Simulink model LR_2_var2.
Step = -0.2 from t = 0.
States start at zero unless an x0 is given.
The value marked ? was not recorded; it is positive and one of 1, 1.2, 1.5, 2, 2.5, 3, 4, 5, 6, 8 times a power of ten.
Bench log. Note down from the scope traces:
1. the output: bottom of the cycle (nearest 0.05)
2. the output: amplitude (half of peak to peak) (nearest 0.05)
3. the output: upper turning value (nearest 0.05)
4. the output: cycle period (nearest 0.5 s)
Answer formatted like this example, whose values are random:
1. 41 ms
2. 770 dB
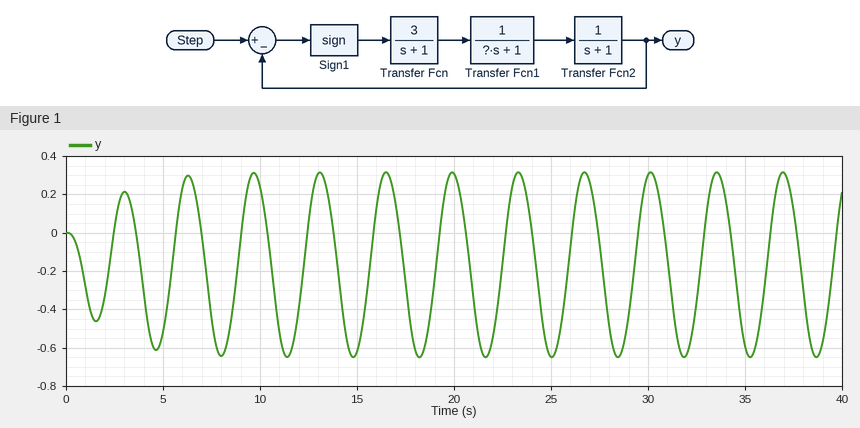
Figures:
1. -0.65
2. 0.50
3. 0.30
4. 3.5 s
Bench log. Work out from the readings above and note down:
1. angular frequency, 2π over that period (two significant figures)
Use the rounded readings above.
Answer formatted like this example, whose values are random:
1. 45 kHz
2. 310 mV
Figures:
1. 1.8 rad/s
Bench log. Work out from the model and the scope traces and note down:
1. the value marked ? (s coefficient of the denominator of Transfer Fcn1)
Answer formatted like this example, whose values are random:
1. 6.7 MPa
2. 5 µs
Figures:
1. 0.8
